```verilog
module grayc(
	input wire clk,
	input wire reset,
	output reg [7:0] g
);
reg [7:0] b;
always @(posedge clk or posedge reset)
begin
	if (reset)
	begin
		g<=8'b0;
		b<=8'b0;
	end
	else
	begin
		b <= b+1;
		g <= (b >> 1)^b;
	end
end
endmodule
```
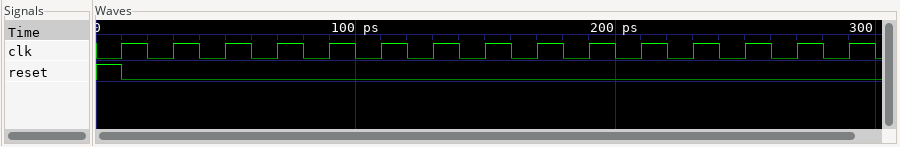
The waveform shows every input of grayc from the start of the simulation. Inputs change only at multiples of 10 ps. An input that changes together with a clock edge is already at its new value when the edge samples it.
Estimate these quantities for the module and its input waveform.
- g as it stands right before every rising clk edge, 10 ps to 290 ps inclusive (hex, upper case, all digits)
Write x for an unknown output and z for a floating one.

00, 00, 01, 03, 02, 06, 07, 05, 04, 0C, 0D, 0F, 0E, 0A, 0B
